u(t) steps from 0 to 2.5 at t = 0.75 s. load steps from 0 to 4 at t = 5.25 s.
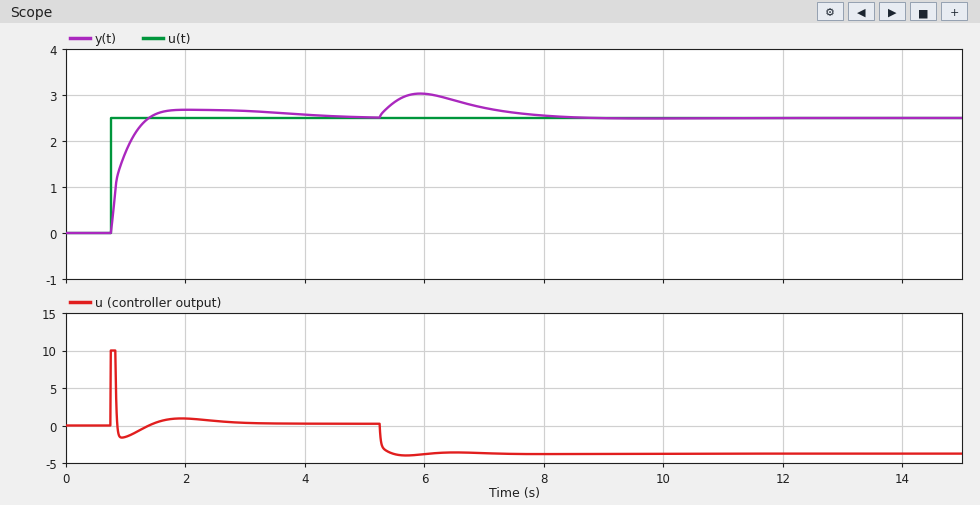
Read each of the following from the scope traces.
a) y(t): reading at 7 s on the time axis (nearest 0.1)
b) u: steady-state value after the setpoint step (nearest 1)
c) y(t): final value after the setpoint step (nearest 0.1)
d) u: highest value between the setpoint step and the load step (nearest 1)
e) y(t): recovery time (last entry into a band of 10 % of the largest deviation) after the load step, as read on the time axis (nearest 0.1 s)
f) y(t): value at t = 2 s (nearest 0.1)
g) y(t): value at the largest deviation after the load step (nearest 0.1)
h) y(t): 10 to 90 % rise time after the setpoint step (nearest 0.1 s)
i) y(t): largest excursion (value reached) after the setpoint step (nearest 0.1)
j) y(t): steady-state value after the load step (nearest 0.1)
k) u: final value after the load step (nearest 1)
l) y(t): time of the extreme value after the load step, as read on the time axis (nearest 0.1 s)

2.7
0
2.5
10
8.0 s
2.7
3.0
0.4 s
2.7
2.5
-4
5.9 s
